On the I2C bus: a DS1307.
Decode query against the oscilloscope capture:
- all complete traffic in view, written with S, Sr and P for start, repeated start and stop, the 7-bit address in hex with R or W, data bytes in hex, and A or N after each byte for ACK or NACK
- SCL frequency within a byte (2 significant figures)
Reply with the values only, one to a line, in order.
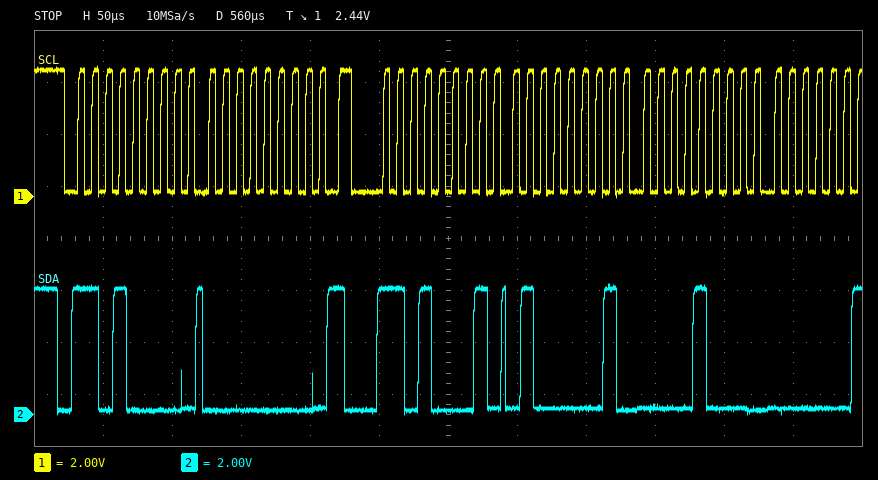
S 68W A 00 A Sr 68R A 41 A 08 A
100 kHz
